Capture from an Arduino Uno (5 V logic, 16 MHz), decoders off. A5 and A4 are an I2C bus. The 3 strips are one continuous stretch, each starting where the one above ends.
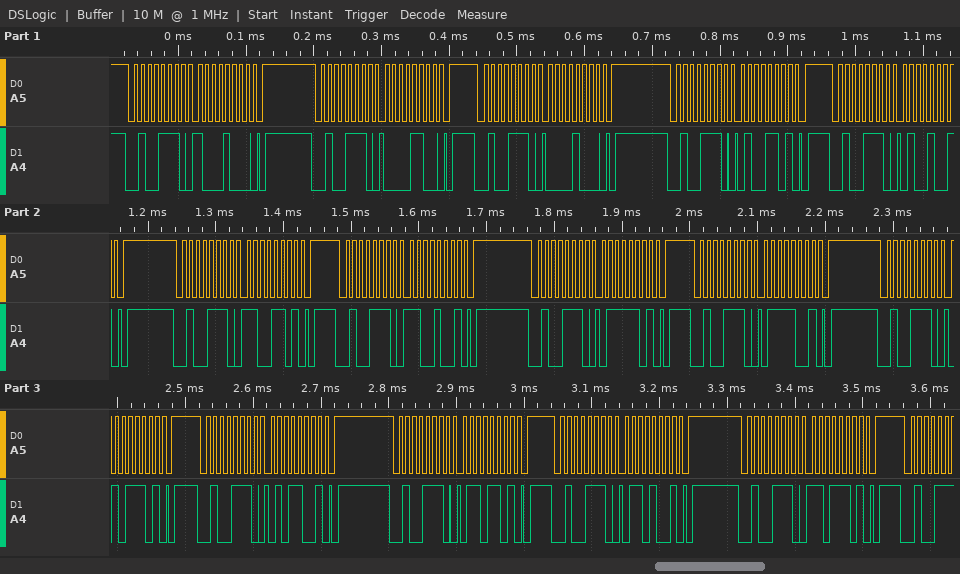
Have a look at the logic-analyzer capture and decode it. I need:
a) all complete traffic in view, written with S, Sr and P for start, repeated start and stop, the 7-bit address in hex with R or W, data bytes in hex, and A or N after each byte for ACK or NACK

S 27W A 88 A P S 27W A 0C A P S 27W A 08 A P S 27W A 4D A P S 27W A 49 A P S 27W A CD A P S 27W A C9 A P S 27W A 7D A P S 27W A 79 A P S 27W A 5D A P S 27W A 59 A P S 27W A 6D A P S 27W A 69 A P S 27W A DD A P
